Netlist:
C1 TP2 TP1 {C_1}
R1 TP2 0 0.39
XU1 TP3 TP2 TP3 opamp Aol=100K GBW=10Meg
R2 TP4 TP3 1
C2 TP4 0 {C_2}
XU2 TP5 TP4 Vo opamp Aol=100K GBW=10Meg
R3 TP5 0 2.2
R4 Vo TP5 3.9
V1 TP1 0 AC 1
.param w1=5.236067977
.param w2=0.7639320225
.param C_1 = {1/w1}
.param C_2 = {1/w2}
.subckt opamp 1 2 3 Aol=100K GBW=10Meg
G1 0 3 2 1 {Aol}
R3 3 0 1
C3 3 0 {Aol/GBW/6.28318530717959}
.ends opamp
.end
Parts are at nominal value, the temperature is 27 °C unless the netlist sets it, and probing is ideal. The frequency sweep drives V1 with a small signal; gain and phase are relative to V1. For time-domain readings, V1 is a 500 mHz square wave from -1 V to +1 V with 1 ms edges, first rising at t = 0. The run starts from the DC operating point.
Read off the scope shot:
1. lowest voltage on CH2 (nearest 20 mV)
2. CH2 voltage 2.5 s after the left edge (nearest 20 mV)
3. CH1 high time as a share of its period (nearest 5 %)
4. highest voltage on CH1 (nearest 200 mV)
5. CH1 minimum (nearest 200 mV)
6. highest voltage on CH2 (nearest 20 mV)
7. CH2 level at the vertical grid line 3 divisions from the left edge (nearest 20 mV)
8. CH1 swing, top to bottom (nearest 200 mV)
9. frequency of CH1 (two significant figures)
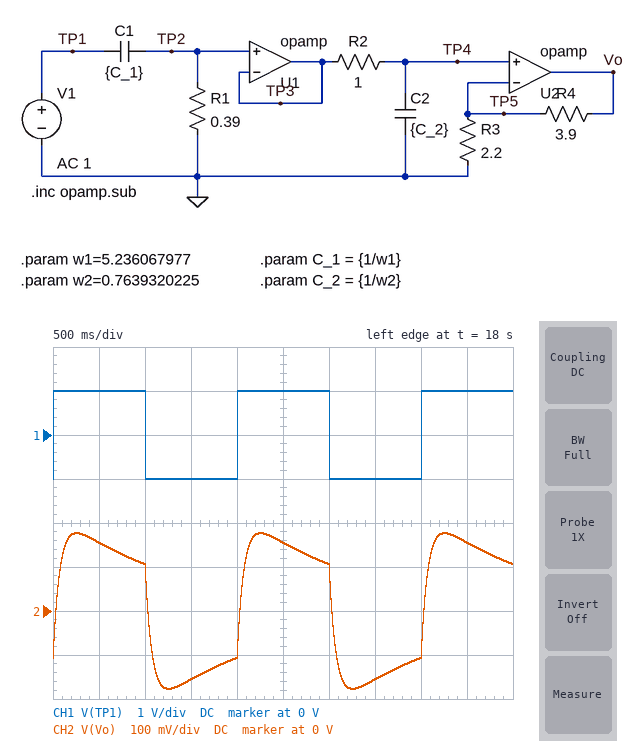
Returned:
-180 mV
160 mV
50 %
1.0 V
-1.0 V
180 mV
-160 mV
2.0 V
500 mHz
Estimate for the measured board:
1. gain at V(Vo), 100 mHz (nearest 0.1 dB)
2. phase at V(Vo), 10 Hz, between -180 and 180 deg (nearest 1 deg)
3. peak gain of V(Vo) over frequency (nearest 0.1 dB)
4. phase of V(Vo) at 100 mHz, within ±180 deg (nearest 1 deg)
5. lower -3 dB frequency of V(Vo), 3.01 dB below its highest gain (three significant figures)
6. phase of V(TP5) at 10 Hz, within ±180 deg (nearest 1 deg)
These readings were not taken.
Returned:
-20.0 dB
-77 deg
-16.5 dB
48 deg
110 mHz
-77 deg
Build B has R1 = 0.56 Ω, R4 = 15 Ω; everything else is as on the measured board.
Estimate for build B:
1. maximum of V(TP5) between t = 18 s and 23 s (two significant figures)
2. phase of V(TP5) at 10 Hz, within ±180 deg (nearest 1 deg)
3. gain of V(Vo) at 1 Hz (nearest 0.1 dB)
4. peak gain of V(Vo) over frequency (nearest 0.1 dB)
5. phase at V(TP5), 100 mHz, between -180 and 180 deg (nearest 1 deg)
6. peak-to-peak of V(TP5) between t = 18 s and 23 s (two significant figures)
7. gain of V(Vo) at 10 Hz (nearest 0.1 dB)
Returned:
86 mV
-81 deg
-5.6 dB
-4.6 dB
47 deg
170 mV
-20.5 dB
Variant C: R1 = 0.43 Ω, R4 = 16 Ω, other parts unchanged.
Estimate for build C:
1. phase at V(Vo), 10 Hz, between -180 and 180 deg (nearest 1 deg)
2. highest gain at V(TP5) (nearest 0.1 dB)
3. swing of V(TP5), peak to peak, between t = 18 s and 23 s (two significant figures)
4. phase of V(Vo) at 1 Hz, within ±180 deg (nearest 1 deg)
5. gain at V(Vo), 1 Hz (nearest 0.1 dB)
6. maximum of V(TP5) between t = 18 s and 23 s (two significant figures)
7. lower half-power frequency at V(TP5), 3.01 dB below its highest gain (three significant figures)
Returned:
-78 deg
-24.6 dB
140 mV
-20 deg
-6.8 dB
69 mV
109 mHz
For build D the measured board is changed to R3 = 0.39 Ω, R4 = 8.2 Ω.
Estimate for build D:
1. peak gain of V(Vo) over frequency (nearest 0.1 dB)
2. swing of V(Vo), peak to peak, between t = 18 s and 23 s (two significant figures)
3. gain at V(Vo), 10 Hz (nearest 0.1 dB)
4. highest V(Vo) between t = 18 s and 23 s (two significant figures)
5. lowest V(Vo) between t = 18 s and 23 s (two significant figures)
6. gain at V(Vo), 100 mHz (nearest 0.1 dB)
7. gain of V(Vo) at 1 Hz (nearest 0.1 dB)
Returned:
1.5 dB
2.8 V
-11.6 dB
1.4 V
-1.4 V
-2.0 dB
1.0 dB
